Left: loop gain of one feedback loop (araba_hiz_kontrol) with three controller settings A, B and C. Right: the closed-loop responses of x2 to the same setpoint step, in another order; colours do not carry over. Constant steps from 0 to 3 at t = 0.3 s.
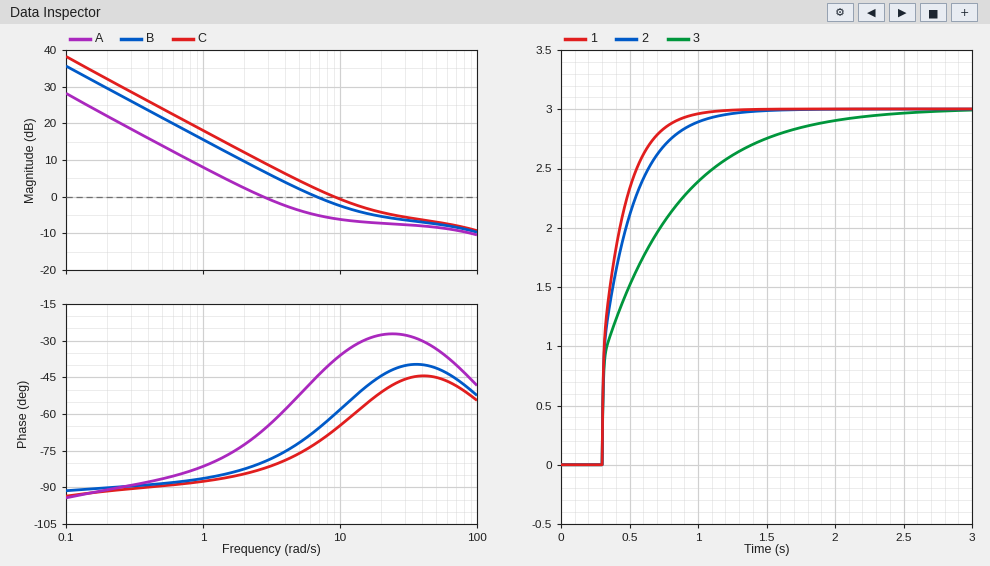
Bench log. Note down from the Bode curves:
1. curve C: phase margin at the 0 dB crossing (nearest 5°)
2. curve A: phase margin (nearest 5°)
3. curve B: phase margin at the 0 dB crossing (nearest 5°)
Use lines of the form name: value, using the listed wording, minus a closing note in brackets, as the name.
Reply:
curve C: phase margin at the 0 dB crossing: 115°
curve A: phase margin: 115°
curve B: phase margin at the 0 dB crossing: 115°
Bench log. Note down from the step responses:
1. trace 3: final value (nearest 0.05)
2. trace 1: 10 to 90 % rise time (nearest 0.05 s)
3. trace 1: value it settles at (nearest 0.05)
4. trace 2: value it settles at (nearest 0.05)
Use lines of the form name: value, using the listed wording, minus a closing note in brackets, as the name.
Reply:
trace 3: final value: 3.00
trace 1: 10 to 90 % rise time: 0.35 s
trace 1: value it settles at: 3.00
trace 2: value it settles at: 3.00
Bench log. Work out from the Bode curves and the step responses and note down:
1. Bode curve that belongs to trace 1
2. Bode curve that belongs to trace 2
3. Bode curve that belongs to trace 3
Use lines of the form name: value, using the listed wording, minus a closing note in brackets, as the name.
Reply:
Bode curve that belongs to trace 1: C
Bode curve that belongs to trace 2: B
Bode curve that belongs to trace 3: A
